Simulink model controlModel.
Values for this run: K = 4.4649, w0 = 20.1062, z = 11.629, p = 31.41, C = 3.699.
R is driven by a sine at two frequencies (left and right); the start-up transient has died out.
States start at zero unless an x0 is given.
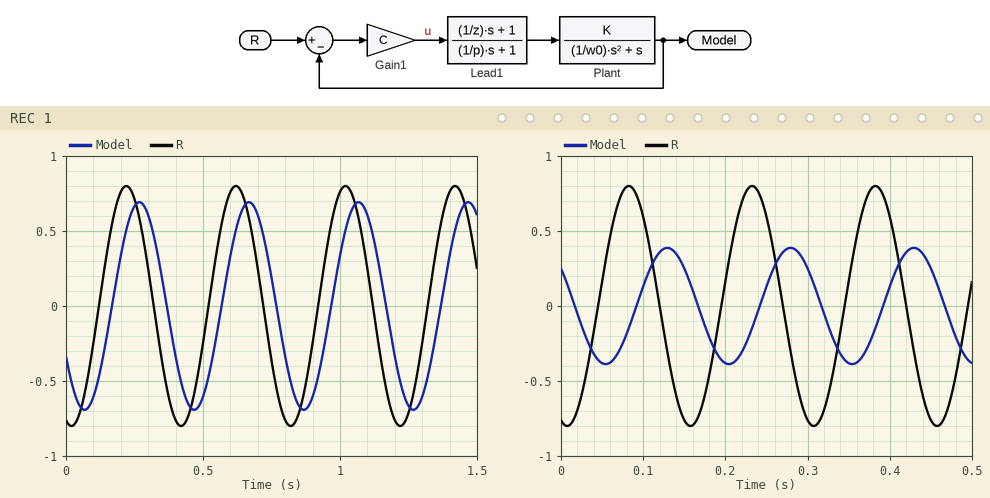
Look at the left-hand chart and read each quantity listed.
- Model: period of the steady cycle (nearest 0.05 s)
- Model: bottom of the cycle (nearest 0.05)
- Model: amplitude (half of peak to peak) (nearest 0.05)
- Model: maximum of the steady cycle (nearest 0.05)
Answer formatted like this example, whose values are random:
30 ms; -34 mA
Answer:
0.40 s; -0.70; 0.70; 0.70
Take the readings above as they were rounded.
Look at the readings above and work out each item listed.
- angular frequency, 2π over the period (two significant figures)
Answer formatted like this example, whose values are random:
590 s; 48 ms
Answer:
16 rad/s
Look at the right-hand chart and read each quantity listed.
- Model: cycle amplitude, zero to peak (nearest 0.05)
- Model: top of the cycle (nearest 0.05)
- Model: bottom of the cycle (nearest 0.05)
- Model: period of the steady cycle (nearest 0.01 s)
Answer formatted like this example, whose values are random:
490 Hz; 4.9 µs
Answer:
0.40; 0.40; -0.40; 0.15 s
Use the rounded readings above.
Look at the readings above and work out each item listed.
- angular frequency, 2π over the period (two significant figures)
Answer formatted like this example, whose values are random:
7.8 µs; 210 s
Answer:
42 rad/s
